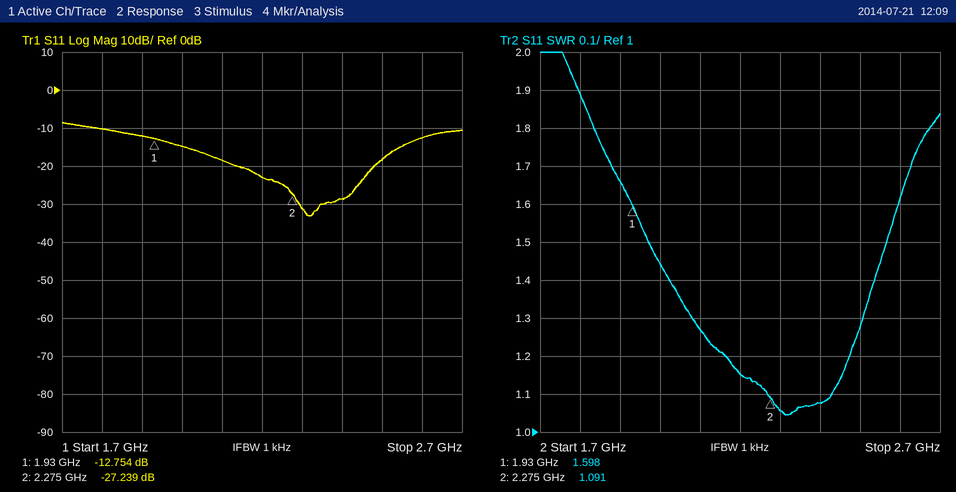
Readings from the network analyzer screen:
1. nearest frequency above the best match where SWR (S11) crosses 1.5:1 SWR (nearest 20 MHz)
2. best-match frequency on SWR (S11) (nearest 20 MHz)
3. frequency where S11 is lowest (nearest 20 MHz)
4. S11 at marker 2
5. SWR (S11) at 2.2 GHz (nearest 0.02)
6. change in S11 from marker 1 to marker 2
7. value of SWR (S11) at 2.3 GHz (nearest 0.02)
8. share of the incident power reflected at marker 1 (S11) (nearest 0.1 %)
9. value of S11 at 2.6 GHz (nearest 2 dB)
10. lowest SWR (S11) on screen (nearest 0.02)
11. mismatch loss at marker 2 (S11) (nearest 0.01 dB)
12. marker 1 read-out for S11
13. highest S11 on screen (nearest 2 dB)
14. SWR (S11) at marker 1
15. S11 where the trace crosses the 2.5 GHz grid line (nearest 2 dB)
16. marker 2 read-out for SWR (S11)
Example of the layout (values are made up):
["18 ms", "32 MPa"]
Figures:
["2.56 GHz", "2.32 GHz", "2.32 GHz", "-27.239 dB", "1.16", "-14.485 dB", "1.06", "5.3 %", "-12 dB", "1.04", "0.01 dB", "-12.754 dB", "-8 dB", "1.598", "-18 dB", "1.091"]
